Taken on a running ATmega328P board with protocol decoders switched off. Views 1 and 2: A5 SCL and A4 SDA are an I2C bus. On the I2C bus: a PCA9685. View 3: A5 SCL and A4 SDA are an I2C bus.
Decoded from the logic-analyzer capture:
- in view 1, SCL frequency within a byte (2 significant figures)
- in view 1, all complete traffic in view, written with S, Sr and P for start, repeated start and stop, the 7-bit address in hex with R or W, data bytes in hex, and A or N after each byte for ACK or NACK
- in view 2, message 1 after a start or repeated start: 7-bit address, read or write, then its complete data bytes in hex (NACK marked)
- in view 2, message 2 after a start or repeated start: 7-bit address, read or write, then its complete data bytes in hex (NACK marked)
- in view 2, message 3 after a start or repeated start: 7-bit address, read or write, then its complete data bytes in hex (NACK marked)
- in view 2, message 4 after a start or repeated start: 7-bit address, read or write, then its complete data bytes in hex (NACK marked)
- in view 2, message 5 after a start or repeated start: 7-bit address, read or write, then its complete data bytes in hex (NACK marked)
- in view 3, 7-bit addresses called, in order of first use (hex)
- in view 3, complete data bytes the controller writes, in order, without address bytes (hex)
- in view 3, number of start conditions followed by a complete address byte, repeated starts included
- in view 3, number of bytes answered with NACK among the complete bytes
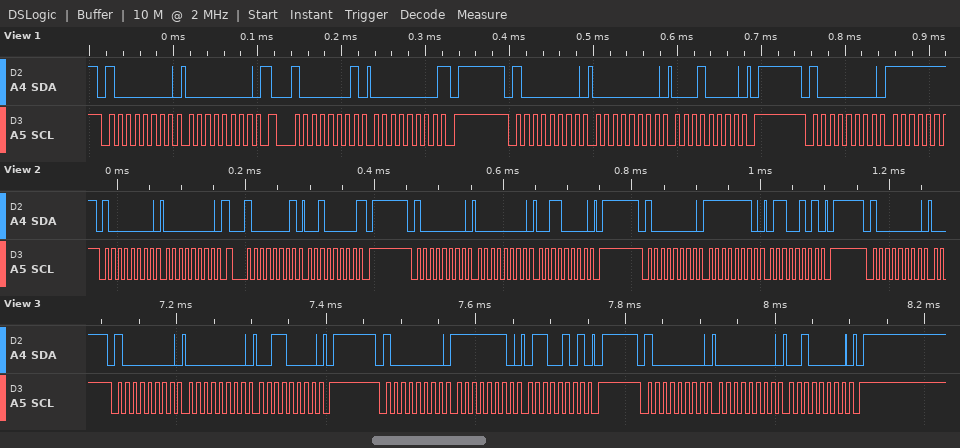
100 kHz
S 40W A 00 A Sr 40R A 00 N P S 40W A 00 A 10 A P S 40W A
0x40 write: 00
0x40 read: 20 NACK
0x40 write: 00 30
0x40 write: FE 65
0x40 write
0x40
00 30 FE 65 00 20
3
0
